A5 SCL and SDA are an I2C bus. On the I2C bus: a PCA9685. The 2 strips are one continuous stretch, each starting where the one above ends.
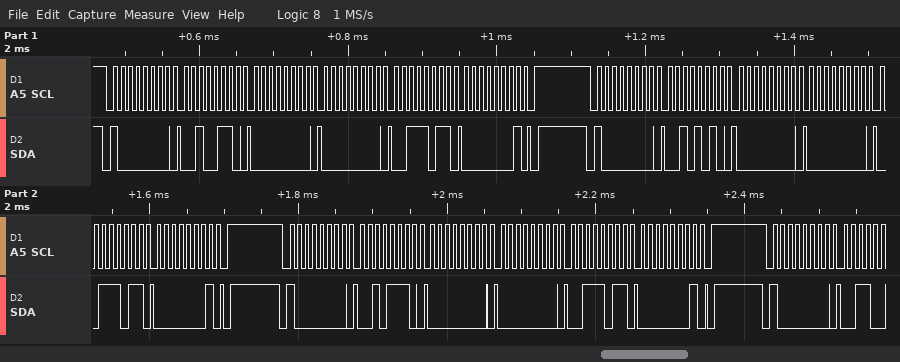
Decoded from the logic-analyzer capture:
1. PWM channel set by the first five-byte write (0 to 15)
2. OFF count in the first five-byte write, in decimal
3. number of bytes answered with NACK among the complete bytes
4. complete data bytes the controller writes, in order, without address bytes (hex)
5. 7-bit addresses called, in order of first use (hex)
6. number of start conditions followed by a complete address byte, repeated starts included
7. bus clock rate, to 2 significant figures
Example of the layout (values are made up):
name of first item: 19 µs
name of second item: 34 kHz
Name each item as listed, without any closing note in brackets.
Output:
PWM channel set by the first five-byte write: 8
OFF count in the first five-byte write, in decimal: 315
number of bytes answered with NACK among the complete bytes: 0
complete data bytes the controller writes, in order, without address bytes: 26 00 00 3B 01 2A 00 00 3B 01 2E 00 00 3B 01
7-bit addresses called, in order of first use: 0x40
number of start conditions followed by a complete address byte, repeated starts included: 4
bus clock rate, to 2 significant figures: 100 kHz
